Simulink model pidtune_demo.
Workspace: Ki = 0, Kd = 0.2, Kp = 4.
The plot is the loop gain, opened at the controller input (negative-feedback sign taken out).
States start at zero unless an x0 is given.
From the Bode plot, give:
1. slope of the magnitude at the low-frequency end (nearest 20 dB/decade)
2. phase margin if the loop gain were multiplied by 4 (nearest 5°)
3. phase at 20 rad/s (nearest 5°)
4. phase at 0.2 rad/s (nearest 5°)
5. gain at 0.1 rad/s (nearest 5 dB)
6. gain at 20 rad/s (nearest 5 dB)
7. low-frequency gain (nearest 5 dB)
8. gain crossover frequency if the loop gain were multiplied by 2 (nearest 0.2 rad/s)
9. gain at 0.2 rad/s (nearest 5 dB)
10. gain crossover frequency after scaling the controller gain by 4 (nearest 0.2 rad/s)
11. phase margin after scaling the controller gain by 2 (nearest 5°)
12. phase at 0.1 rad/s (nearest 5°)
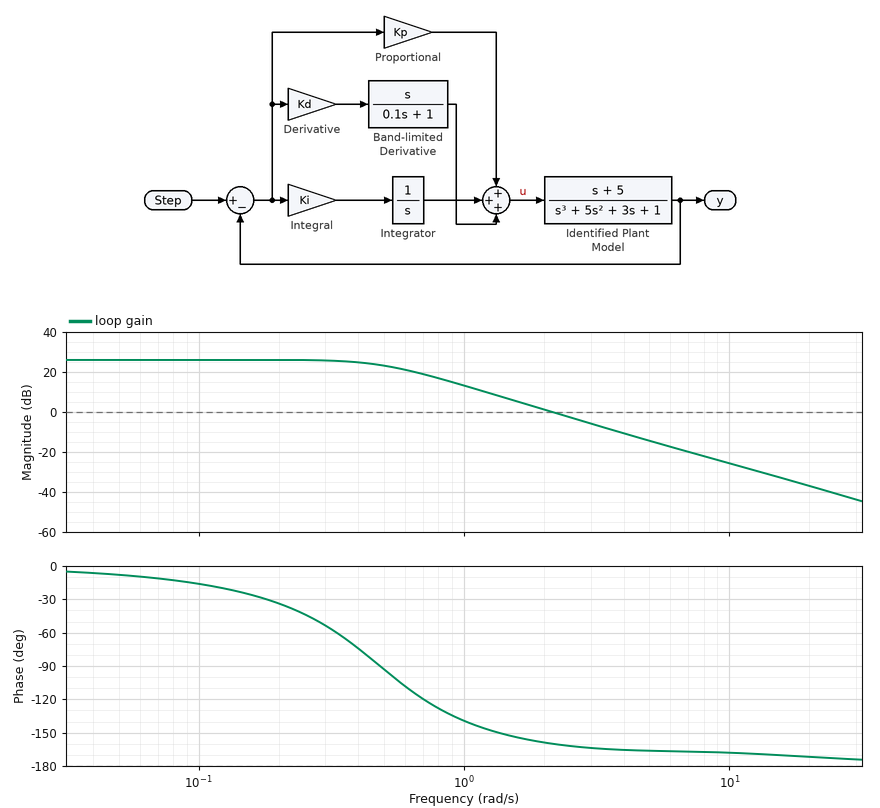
0 dB/decade
15°
-170°
-35°
25 dB
-35 dB
25 dB
3.0 rad/s
25 dB
4.4 rad/s
15°
-15°
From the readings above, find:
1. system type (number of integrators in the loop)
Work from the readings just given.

0
